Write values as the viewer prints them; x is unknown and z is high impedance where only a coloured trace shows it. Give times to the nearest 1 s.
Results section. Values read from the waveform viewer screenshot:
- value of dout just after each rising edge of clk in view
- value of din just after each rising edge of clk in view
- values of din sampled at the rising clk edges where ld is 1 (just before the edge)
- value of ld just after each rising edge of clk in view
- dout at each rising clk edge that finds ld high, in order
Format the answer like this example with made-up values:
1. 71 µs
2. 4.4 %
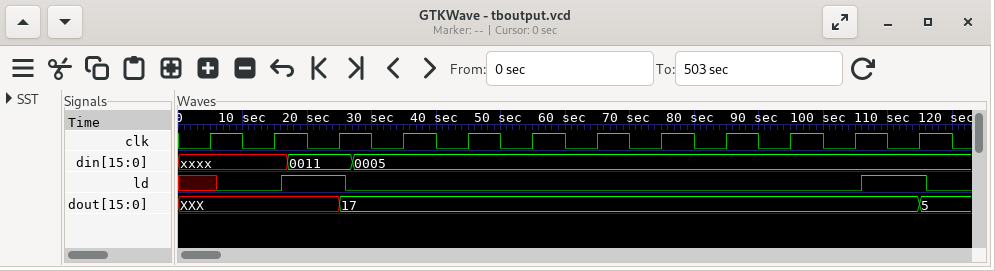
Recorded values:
1. XXX, XXX, 17, 17, 17, 17, 17, 17, 17, 17, 17, 5
2. xxxx, xxxx, 0011, 0005, 0005, 0005, 0005, 0005, 0005, 0005, 0005, 0005
3. 0011, 0005
4. x 0 1 0 0 0 0 0 0 0 0 1
5. XXX, 17
